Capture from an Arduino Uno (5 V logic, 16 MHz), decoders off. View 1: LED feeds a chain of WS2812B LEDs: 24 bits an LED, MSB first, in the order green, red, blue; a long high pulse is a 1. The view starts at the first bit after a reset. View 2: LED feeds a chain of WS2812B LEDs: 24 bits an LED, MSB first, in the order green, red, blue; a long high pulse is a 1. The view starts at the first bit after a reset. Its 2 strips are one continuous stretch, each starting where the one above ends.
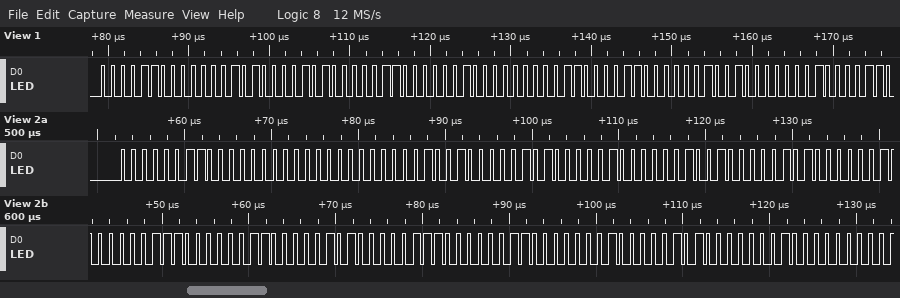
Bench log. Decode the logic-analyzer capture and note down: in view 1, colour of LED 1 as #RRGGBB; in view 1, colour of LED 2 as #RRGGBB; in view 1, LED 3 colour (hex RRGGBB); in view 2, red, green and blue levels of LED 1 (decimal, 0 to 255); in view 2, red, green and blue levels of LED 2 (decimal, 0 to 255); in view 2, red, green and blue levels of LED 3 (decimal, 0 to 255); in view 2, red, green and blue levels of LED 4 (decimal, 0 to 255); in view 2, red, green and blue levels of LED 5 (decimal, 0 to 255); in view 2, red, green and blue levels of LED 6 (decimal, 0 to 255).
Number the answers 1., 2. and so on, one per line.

1. #050C0A
2. #080C03
3. #090C01
4. 0, 3, 0
5. 5, 9, 4
6. 5, 9, 2
7. 3, 7, 5
8. 3, 7, 1
9. 1, 5, 0
